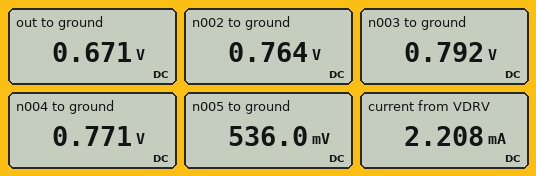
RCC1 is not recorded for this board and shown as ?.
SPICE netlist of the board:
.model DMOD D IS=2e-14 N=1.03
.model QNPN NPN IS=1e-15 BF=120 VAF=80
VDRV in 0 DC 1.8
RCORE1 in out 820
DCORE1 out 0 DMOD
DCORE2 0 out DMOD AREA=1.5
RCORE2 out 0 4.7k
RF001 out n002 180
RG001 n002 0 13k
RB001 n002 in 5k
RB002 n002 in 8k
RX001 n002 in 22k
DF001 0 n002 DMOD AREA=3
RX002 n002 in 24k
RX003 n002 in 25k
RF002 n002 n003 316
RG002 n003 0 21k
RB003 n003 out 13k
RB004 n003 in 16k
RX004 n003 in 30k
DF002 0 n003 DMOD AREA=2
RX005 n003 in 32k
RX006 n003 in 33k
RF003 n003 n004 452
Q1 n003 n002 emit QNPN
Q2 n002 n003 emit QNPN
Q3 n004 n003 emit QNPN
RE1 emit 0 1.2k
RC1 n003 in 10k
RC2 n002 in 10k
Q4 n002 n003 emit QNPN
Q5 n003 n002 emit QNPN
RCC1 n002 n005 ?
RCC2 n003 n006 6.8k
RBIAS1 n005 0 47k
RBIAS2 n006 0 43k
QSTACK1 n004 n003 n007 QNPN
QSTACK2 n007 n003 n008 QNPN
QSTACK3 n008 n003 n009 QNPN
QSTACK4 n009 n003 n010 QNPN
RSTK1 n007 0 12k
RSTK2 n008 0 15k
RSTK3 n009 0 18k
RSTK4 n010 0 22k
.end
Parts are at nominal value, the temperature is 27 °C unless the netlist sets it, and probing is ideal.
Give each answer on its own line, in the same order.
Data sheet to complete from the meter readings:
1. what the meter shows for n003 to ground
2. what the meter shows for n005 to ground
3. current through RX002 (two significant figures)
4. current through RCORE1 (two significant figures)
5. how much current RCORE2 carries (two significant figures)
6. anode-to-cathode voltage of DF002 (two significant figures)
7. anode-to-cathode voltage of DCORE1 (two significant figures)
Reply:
0.792 V
536.0 mV
43 µA
1.4 mA
140 µA
-790 mV
670 mV
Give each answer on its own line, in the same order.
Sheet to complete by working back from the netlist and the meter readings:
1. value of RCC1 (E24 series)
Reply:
20 kΩ
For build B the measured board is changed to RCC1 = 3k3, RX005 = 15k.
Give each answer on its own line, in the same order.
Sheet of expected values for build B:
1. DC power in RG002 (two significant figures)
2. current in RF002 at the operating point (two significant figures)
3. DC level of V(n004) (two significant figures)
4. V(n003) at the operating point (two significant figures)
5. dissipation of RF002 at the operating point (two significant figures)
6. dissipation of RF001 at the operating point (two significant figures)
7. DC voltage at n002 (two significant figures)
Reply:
31 µW
120 µA
780 mV
800 mV
4.2 µW
51 µW
770 mV
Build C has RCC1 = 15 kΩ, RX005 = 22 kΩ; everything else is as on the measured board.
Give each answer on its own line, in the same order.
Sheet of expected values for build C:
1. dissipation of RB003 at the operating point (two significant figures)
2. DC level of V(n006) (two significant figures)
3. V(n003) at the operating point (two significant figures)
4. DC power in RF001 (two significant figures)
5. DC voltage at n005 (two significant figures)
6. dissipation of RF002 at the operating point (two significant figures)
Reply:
1.2 µW
690 mV
800 mV
49 µW
580 mV
3.1 µW
